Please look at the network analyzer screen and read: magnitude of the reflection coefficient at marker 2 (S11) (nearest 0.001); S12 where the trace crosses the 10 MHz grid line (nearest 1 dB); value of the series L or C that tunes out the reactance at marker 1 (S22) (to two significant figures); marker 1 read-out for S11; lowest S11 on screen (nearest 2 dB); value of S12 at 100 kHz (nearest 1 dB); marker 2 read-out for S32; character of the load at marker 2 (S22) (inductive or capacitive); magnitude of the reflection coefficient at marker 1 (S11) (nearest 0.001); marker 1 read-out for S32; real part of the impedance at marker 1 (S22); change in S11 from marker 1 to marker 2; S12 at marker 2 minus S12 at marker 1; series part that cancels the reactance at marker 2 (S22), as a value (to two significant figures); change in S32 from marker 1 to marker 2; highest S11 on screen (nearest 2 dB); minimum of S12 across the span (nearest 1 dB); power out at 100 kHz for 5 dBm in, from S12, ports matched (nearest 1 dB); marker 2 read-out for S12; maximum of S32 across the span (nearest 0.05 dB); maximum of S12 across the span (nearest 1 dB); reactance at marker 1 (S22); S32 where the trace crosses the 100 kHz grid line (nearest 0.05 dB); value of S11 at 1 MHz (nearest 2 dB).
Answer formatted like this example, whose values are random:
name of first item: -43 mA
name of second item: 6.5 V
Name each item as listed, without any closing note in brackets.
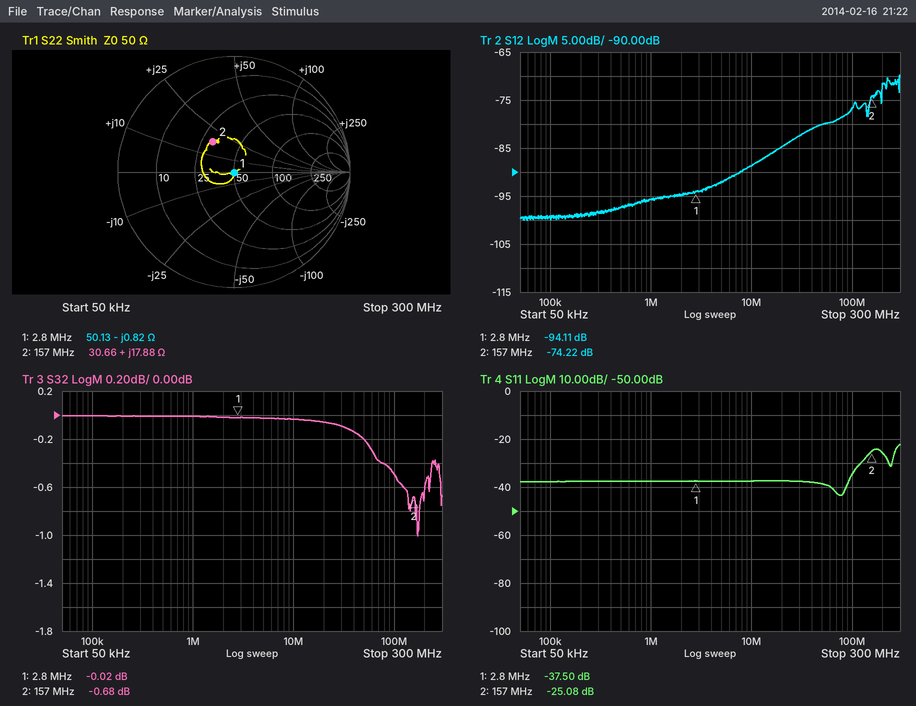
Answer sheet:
magnitude of the reflection coefficient at marker 2 (S11): 0.056
S12 where the trace crosses the 10 MHz grid line: -89 dB
value of the series L or C that tunes out the reactance at marker 1 (S22): 47 nH
marker 1 read-out for S11: -37.50 dB
lowest S11 on screen: -44 dB
value of S12 at 100 kHz: -99 dB
marker 2 read-out for S32: -0.68 dB
character of the load at marker 2 (S22): inductive
magnitude of the reflection coefficient at marker 1 (S11): 0.013
marker 1 read-out for S32: -0.02 dB
real part of the impedance at marker 1: 50.13 Ω
change in S11 from marker 1 to marker 2: 12.42 dB
S12 at marker 2 minus S12 at marker 1: 19.89 dB
series part that cancels the reactance at marker 2 (S22), as a value: 57 pF
change in S32 from marker 1 to marker 2: -0.66 dB
highest S11 on screen: -22 dB
minimum of S12 across the span: -100 dB
power out at 100 kHz for 5 dBm in, from S12, ports matched: -94 dBm
marker 2 read-out for S12: -74.22 dB
maximum of S32 across the span: 0.00 dB
maximum of S12 across the span: -70 dB
reactance at marker 1: -0.82 Ω
S32 where the trace crosses the 100 kHz grid line: 0.00 dB
value of S11 at 1 MHz: -38 dB
